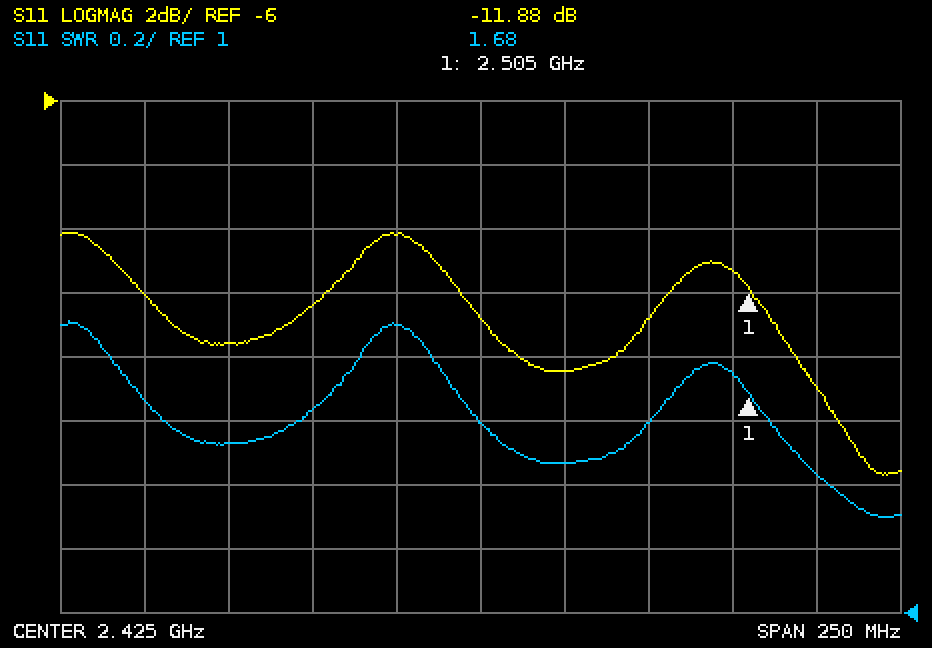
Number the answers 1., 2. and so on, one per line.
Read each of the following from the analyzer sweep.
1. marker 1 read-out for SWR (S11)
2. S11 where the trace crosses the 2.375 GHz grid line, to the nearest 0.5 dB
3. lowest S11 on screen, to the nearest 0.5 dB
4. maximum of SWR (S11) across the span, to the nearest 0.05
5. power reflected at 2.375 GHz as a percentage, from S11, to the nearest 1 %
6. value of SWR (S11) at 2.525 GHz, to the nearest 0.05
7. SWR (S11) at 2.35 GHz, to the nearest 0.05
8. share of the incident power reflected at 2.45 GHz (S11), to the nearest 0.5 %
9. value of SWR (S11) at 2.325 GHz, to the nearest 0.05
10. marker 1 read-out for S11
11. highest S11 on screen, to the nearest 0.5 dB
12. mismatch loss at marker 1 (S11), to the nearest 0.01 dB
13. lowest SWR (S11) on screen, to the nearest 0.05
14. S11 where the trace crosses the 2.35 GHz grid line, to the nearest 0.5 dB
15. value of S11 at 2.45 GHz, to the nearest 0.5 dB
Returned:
1. 1.68
2. -12.5 dB
3. -17.5 dB
4. 1.90
5. 6 %
6. 1.45
7. 1.55
8. 3.5 %
9. 1.65
10. -11.88 dB
11. -10.0 dB
12. 0.29 dB
13. 1.30
14. -13.5 dB
15. -14.5 dB
